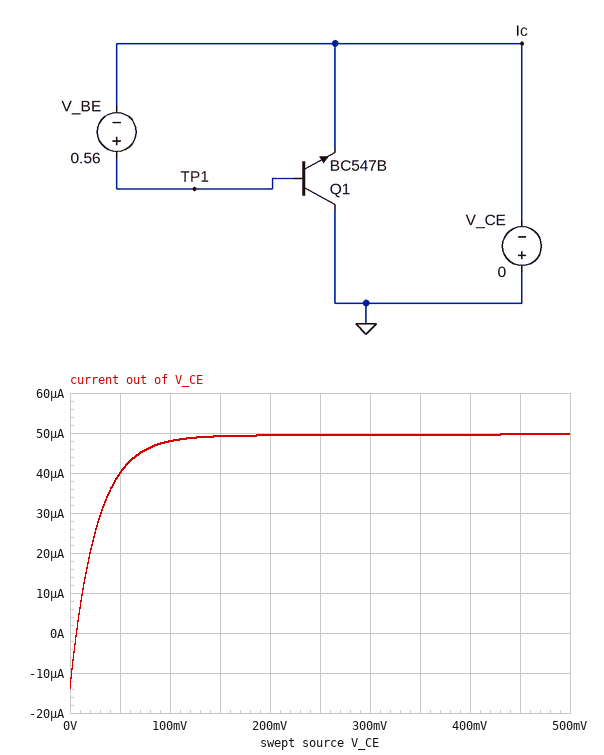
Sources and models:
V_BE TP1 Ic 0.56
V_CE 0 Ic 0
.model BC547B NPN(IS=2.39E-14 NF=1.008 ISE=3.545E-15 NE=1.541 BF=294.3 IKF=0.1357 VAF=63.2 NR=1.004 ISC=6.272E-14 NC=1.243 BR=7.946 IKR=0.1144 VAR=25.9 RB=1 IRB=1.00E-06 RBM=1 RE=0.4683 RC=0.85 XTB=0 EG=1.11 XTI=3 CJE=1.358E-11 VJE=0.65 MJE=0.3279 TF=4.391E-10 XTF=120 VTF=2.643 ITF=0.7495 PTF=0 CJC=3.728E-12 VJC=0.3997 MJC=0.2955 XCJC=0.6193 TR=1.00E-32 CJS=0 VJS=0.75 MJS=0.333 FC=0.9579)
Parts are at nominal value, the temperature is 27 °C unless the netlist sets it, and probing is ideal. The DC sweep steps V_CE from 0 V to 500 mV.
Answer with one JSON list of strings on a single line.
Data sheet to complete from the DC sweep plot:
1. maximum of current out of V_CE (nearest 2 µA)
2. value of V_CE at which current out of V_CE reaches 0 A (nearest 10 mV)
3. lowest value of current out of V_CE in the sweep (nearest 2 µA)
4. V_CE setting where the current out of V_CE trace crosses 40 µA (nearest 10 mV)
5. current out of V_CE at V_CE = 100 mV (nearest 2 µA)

["50 µA", "10 mV", "-14 µA", "50 mV", "48 µA"]
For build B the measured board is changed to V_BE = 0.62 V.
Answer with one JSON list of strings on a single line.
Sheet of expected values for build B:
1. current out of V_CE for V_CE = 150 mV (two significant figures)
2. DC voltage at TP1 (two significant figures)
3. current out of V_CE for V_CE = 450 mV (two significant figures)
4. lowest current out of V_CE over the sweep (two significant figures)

["480 µA", "620 mV", "490 µA", "-130 µA"]
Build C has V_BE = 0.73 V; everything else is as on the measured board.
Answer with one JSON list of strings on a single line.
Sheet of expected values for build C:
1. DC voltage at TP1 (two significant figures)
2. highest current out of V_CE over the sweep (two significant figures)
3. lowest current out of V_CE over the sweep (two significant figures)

["730 mV", "20 mA", "-3.8 mA"]
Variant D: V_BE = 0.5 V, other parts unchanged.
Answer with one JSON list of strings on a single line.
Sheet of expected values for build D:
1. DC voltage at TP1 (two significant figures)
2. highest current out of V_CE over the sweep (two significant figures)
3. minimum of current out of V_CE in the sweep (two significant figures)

["500 mV", "5.0 µA", "-1.4 µA"]
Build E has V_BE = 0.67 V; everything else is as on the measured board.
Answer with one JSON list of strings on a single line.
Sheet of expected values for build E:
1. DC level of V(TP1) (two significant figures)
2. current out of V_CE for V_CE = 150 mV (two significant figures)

["670 mV", "3.1 mA"]
